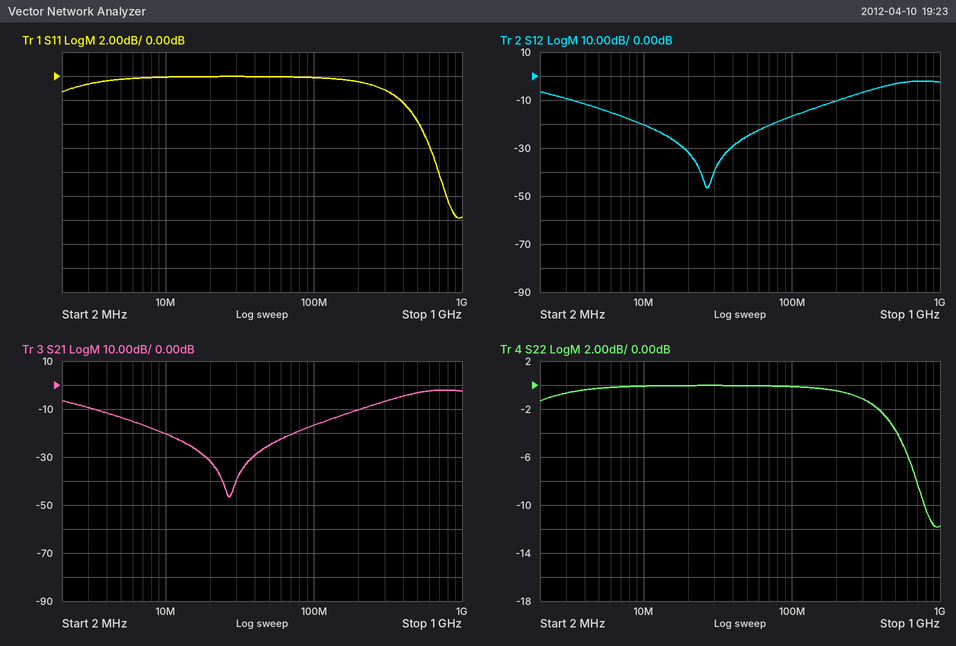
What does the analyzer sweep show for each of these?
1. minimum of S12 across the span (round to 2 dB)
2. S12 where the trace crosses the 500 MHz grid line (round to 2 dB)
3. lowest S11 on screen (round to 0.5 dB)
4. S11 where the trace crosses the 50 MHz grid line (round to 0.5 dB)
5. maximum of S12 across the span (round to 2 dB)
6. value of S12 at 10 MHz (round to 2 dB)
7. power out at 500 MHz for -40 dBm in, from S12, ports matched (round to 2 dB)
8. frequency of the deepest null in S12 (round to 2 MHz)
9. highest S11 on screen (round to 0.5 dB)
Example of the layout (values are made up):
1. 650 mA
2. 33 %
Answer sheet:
1. -46 dB
2. -4 dB
3. -12.0 dB
4. 0.0 dB
5. -2 dB
6. -20 dB
7. -44 dBm
8. 26 MHz
9. 0.0 dB
